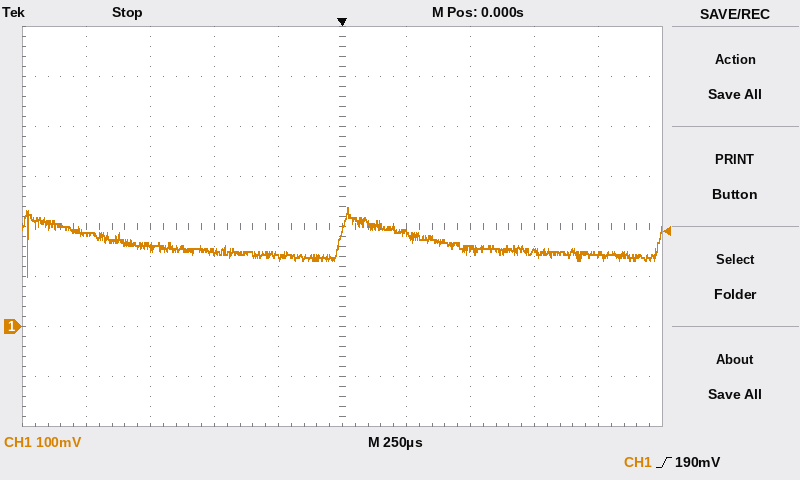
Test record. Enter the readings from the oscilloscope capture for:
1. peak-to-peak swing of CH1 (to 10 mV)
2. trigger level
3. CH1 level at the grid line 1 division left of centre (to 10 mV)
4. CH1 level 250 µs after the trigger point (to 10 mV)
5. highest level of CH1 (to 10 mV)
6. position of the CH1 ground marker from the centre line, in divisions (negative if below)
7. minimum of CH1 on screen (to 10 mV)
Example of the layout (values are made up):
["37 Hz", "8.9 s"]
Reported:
["140 mV", "190 mV", "140 mV", "190 mV", "240 mV", "-2.0 div", "100 mV"]
